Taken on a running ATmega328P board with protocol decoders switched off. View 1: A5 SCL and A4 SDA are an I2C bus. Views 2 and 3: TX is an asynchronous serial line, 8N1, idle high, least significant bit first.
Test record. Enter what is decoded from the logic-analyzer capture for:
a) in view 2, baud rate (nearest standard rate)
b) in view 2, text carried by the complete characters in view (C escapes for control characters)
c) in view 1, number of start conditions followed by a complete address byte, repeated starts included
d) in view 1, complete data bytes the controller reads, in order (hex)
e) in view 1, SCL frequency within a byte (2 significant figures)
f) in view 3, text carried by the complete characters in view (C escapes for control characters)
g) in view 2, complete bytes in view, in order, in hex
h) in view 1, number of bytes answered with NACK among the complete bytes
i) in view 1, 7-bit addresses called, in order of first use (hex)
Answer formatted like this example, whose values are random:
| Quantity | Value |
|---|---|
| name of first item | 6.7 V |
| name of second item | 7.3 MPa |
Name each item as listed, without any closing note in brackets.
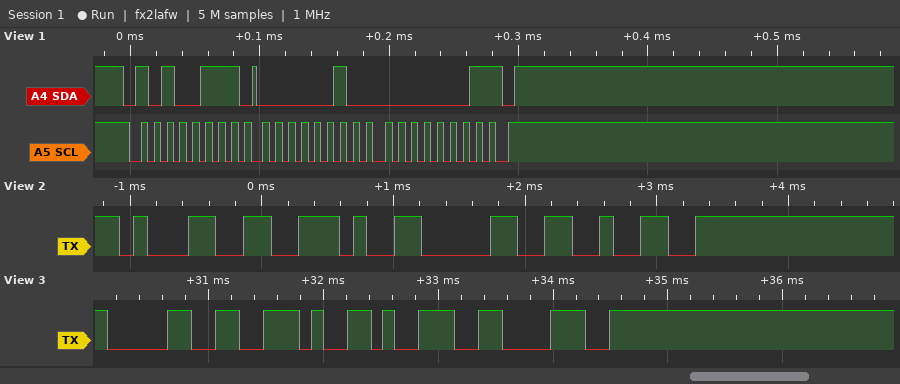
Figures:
| Quantity | Value |
|---|---|
| in view 2, baud rate | 9600 baud |
| in view 2, text carried by the complete characters in view | "1.02" |
| in view 1, number of start conditions followed by a complete address byte, repeated starts included | 1 |
| in view 1, complete data bytes the controller reads, in order | 02 01 |
| in view 1, SCL frequency within a byte | 100 kHz |
| in view 3, text carried by the complete characters in view | "0.98" |
| in view 2, complete bytes in view, in order, in hex | 31 2E 30 32 |
| in view 1, number of bytes answered with NACK among the complete bytes | 1 |
| in view 1, 7-bit addresses called, in order of first use | 0x53 |
